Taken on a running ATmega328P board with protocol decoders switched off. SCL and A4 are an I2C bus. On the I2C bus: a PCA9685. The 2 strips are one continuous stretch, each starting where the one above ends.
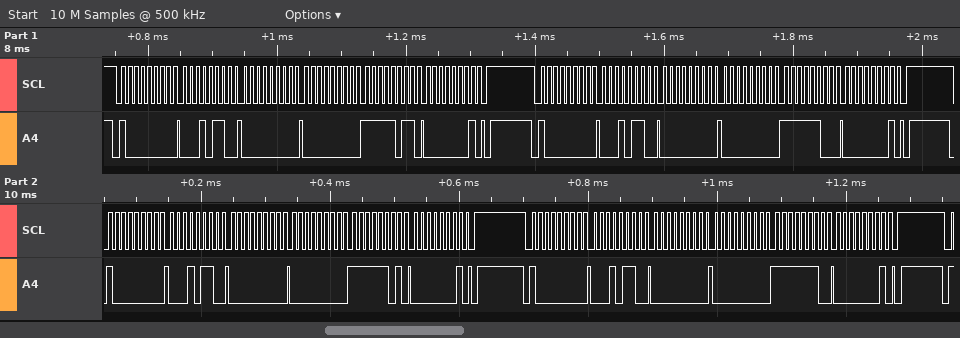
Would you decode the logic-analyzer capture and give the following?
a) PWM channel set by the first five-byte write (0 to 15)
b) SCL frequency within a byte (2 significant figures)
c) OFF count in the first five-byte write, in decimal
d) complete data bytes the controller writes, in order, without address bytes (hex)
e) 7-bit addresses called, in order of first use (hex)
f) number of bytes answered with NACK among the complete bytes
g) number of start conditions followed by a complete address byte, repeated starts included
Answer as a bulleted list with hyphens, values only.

- 4
- 100 kHz
- 507
- 16 00 00 FB 01 16 00 00 FC 01 16 00 00 FD 01 16 00 00 FE 01
- 0x40
- 0
- 4
